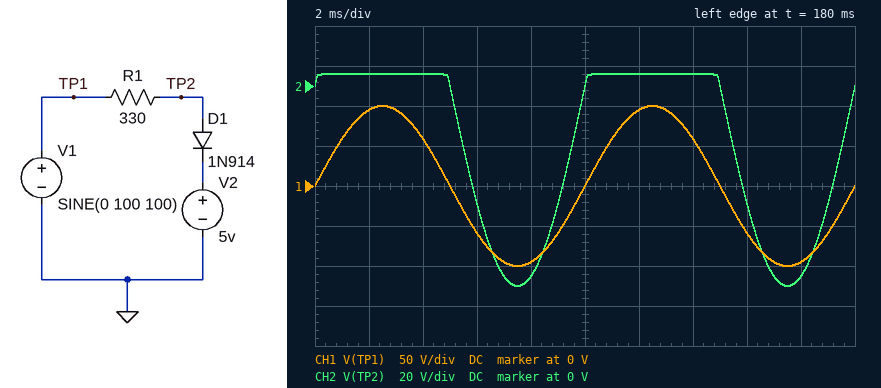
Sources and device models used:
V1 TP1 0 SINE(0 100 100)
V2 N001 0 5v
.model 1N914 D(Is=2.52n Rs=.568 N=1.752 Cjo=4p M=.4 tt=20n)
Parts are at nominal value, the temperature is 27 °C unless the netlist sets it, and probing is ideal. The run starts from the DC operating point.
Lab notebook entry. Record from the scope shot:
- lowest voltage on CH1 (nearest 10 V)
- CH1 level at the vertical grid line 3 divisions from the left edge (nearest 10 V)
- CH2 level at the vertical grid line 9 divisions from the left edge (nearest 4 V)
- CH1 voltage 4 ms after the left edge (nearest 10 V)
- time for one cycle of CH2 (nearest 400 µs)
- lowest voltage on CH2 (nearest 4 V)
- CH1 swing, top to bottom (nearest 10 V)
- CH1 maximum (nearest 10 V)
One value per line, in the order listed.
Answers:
-100 V
-60 V
-96 V
60 V
10.0 ms
-100 V
200 V
100 V
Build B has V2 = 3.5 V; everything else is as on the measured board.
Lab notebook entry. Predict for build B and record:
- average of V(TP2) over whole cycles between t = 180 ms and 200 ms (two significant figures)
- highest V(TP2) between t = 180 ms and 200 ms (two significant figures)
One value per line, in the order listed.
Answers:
-30 V
4.5 V
